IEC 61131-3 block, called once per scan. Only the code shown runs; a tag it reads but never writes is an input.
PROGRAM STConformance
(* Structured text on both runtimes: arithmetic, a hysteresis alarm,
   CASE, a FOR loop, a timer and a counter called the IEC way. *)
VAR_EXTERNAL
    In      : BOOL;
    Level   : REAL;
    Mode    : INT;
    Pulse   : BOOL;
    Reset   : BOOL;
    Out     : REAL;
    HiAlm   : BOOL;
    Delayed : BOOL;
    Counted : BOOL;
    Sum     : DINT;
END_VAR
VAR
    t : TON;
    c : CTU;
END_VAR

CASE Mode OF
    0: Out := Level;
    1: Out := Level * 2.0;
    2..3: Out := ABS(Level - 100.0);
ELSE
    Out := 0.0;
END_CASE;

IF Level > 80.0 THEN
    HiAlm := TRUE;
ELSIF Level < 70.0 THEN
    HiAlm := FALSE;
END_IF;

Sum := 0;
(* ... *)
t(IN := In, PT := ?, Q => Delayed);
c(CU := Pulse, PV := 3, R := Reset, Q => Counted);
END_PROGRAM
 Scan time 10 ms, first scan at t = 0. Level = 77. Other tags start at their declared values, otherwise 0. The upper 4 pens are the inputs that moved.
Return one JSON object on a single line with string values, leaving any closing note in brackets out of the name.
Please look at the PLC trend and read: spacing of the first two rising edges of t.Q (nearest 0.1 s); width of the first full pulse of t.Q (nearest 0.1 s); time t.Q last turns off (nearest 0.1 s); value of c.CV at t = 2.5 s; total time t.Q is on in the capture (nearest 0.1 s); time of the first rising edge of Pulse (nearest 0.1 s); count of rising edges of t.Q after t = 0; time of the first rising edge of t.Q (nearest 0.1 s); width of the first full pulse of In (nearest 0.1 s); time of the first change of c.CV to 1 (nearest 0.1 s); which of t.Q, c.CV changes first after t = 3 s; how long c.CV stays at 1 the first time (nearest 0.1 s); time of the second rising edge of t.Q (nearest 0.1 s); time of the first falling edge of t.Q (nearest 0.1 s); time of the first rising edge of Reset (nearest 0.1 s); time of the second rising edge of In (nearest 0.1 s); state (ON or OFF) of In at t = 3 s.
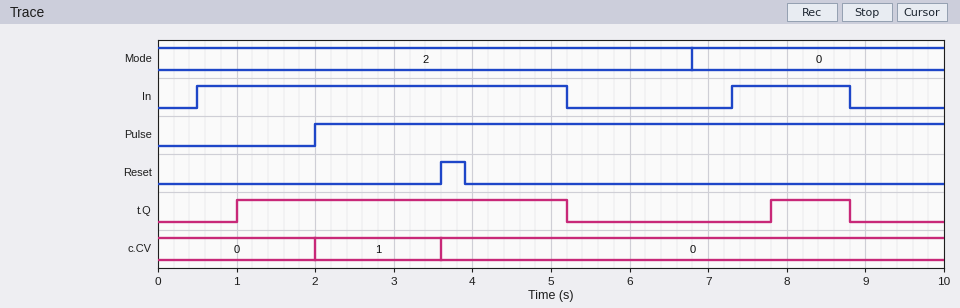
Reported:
{"spacing of the first two rising edges of t.Q": "6.8 s", "width of the first full pulse of t.Q": "4.2 s", "time t.Q last turns off": "8.8 s", "value of c.CV at t = 2.5 s": "1", "total time t.Q is on in the capture": "5.2 s", "time of the first rising edge of Pulse": "2.0 s", "count of rising edges of t.Q after t = 0": "2", "time of the first rising edge of t.Q": "1.0 s", "width of the first full pulse of In": "4.7 s", "time of the first change of c.CV to 1": "2.0 s", "which of t.Q, c.CV changes first after t = 3 s": "c.CV", "how long c.CV stays at 1 the first time": "1.6 s", "time of the second rising edge of t.Q": "7.8 s", "time of the first falling edge of t.Q": "5.2 s", "time of the first rising edge of Reset": "3.6 s", "time of the second rising edge of In": "7.3 s", "state (ON or OFF) of In at t = 3 s": "ON"}
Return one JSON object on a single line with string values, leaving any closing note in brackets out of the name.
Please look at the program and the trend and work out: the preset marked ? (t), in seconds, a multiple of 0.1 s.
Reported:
{"the preset marked ? (t), in seconds, a multiple of 0.1 s": "0.5 s"}
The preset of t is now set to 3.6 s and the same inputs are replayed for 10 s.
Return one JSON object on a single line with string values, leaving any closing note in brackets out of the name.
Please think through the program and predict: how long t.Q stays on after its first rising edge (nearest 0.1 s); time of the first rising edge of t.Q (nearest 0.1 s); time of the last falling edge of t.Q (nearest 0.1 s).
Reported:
{"how long t.Q stays on after its first rising edge": "1.1 s", "time of the first rising edge of t.Q": "4.1 s", "time of the last falling edge of t.Q": "5.2 s"}
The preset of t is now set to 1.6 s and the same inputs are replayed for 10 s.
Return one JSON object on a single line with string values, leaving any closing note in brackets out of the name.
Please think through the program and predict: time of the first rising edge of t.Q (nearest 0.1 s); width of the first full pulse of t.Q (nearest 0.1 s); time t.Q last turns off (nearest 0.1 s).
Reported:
{"time of the first rising edge of t.Q": "2.1 s", "width of the first full pulse of t.Q": "3.1 s", "time t.Q last turns off": "5.2 s"}
